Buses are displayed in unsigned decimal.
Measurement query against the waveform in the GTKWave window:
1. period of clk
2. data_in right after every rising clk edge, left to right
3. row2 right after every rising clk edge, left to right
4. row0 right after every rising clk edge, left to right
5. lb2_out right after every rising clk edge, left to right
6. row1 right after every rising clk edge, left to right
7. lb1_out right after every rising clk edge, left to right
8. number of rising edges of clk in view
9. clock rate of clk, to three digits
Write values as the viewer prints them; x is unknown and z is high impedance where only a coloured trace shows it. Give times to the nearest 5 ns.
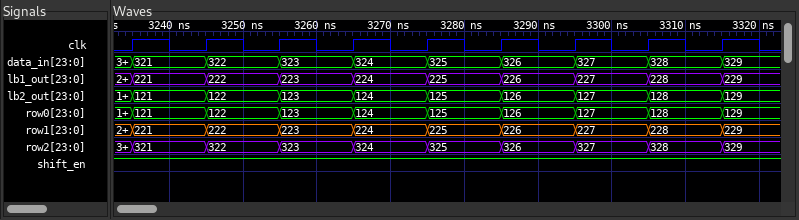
10 ns
321, 322, 323, 324, 325, 326, 327, 328, 329
321, 322, 323, 324, 325, 326, 327, 328, 329
121, 122, 123, 124, 125, 126, 127, 128, 129
121, 122, 123, 124, 125, 126, 127, 128, 129
221, 222, 223, 224, 225, 226, 227, 228, 229
221, 222, 223, 224, 225, 226, 227, 228, 229
9
100 MHz
